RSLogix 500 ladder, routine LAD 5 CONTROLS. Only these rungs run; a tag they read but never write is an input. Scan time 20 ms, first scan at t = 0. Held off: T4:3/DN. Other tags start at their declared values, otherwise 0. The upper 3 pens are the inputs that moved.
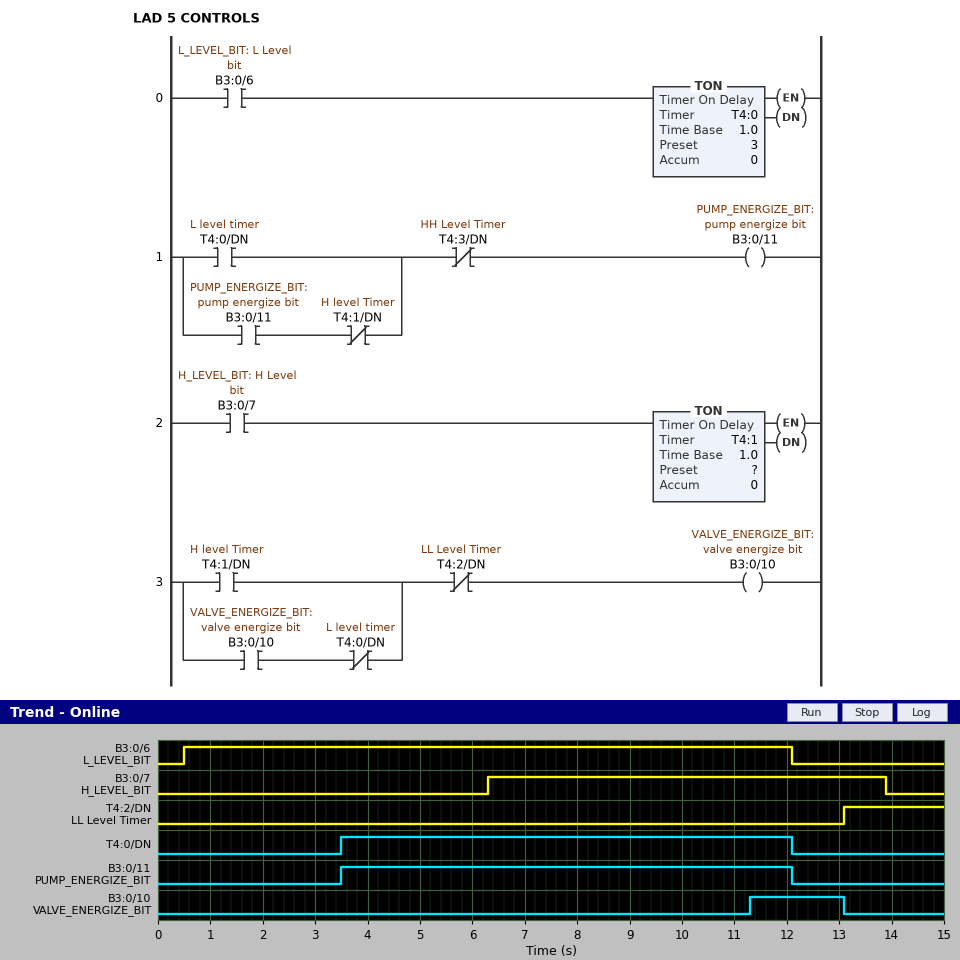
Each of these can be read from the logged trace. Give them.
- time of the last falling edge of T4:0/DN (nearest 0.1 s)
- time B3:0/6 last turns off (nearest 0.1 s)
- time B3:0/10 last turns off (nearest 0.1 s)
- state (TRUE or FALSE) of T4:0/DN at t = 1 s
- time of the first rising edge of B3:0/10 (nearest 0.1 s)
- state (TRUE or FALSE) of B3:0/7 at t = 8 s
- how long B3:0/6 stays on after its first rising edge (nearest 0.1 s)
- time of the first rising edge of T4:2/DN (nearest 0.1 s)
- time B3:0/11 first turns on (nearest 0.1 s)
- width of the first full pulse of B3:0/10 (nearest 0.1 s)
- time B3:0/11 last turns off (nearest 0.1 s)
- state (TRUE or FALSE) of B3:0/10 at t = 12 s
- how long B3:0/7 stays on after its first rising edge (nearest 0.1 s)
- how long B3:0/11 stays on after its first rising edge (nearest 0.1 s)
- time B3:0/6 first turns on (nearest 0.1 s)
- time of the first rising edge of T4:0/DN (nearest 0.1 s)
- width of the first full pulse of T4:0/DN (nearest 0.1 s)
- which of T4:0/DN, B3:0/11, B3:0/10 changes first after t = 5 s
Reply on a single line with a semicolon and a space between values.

12.1 s; 12.1 s; 13.1 s; FALSE; 11.3 s; TRUE; 11.6 s; 13.1 s; 3.5 s; 1.8 s; 12.1 s; TRUE; 7.6 s; 8.6 s; 0.5 s; 3.5 s; 8.6 s; B3:0/10
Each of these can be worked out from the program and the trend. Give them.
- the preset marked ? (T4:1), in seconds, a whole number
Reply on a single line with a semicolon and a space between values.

5 s
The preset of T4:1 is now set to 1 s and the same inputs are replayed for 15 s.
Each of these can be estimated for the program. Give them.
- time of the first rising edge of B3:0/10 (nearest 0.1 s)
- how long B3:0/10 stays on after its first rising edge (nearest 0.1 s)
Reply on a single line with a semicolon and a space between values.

7.3 s; 5.8 s
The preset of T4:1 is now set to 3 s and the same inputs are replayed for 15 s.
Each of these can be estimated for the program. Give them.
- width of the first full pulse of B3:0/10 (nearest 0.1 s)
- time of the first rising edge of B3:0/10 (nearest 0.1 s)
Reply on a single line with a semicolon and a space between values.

3.8 s; 9.3 s
